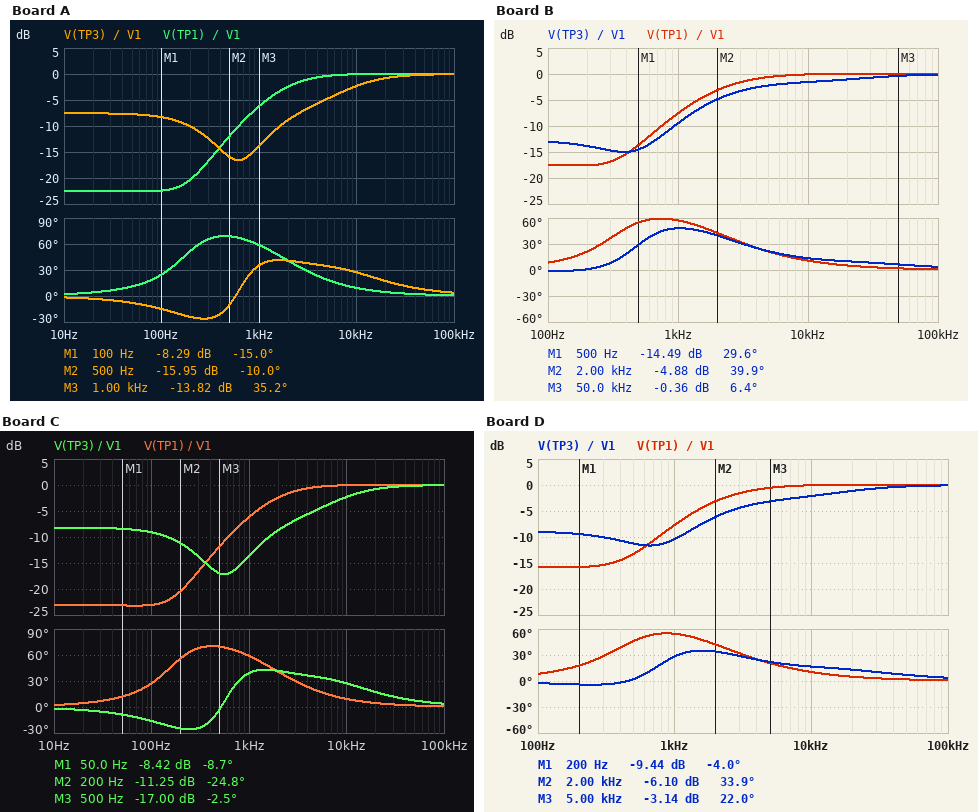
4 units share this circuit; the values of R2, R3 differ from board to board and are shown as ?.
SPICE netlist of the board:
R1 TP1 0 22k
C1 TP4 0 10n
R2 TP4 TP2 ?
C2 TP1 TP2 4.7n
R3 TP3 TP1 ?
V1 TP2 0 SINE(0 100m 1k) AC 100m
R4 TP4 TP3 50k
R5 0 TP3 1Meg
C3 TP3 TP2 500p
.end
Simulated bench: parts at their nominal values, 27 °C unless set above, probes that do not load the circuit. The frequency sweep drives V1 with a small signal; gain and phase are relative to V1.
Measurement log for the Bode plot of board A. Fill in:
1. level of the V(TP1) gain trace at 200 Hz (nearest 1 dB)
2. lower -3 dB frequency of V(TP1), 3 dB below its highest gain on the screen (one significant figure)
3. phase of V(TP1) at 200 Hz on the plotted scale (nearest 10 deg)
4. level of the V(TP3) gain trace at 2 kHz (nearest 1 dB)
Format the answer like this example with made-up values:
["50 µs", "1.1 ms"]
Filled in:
["-20 dB", "2 kHz", "50 deg", "-9 dB"]
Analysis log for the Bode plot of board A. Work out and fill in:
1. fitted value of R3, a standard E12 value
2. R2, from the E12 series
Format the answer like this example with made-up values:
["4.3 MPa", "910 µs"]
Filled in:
["100 kΩ", "100 kΩ"]
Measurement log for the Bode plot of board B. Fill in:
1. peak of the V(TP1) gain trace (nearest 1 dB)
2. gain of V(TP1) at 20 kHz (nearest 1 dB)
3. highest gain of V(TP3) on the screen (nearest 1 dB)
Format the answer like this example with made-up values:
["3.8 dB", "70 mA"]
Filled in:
["0 dB", "0 dB", "0 dB"]
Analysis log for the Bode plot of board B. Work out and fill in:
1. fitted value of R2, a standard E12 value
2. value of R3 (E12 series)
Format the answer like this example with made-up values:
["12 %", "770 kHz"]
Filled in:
["68 kΩ", "15 kΩ"]
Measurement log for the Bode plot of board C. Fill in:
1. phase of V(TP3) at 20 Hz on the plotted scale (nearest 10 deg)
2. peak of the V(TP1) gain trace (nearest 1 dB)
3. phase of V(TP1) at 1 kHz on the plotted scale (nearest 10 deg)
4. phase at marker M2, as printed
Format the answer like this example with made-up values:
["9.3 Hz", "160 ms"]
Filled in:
["0 deg", "0 dB", "60 deg", "-24.8 deg"]
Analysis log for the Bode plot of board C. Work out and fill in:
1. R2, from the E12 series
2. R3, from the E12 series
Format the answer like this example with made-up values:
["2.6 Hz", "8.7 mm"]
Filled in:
["120 kΩ", "100 kΩ"]
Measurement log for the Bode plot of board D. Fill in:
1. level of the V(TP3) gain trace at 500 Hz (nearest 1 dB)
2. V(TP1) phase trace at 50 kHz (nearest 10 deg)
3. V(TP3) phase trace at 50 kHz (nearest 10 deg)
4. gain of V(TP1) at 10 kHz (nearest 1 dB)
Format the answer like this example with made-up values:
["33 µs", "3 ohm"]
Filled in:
["-11 dB", "0 deg", "10 deg", "0 dB"]
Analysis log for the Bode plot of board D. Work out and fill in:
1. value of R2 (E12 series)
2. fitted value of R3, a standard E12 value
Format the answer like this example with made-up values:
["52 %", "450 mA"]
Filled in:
["33 kΩ", "27 kΩ"]
